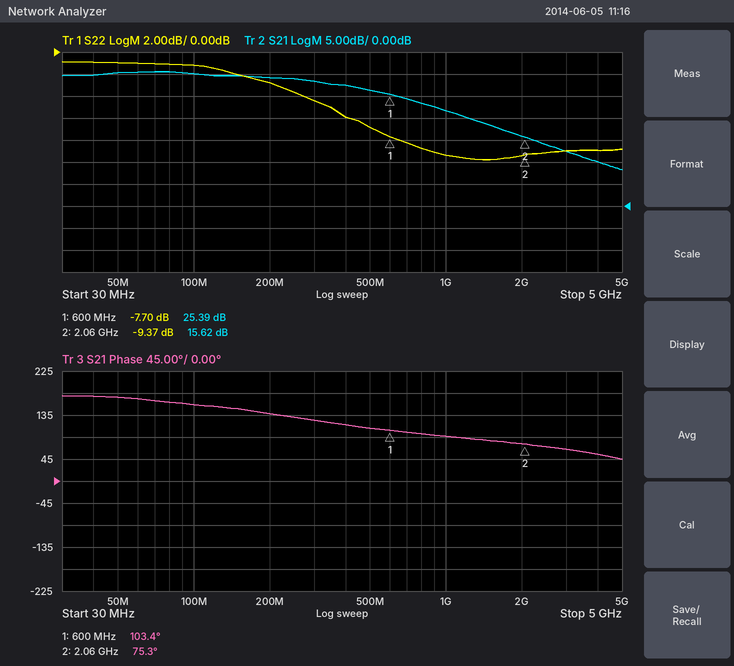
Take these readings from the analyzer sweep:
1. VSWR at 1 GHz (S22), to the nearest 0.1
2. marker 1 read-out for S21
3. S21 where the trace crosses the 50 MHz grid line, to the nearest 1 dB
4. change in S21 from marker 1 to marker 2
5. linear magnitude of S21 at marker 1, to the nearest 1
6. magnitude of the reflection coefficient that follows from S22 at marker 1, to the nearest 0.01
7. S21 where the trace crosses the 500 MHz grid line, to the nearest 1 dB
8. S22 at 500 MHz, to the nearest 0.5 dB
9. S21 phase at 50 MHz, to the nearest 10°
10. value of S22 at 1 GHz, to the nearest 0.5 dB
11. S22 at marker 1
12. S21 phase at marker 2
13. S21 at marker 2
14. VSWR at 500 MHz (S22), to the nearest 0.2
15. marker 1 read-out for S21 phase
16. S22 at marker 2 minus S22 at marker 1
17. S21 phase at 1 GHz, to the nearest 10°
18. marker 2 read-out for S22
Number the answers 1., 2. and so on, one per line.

1. 2.0
2. 25.39 dB
3. 30 dB
4. -9.77 dB
5. 19
6. 0.41
7. 26 dB
8. -7.0 dB
9. 170°
10. -9.5 dB
11. -7.70 dB
12. 75.3°
13. 15.62 dB
14. 2.6
15. 103.4°
16. -1.67 dB
17. 90°
18. -9.37 dB
